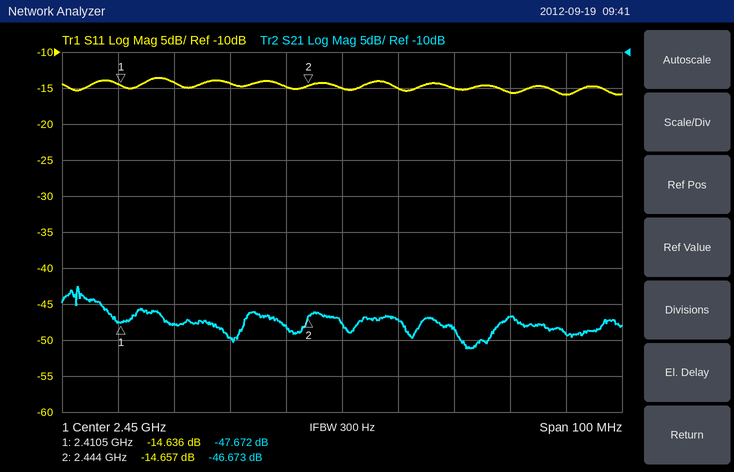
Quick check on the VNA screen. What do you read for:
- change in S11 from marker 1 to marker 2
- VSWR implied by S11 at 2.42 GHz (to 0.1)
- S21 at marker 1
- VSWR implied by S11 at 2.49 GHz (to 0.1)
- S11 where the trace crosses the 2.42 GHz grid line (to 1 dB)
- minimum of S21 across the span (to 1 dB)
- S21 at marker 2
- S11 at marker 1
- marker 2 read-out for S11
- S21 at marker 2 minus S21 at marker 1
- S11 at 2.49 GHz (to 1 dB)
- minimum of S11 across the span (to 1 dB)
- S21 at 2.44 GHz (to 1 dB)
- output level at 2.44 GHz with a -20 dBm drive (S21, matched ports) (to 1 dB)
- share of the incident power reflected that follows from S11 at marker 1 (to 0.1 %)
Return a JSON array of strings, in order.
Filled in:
["-0.021 dB", "1.5", "-47.672 dB", "1.4", "-14 dB", "-51 dB", "-46.673 dB", "-14.636 dB", "-14.657 dB", "0.999 dB", "-16 dB", "-16 dB", "-48 dB", "-68 dBm", "3.4 %"]
